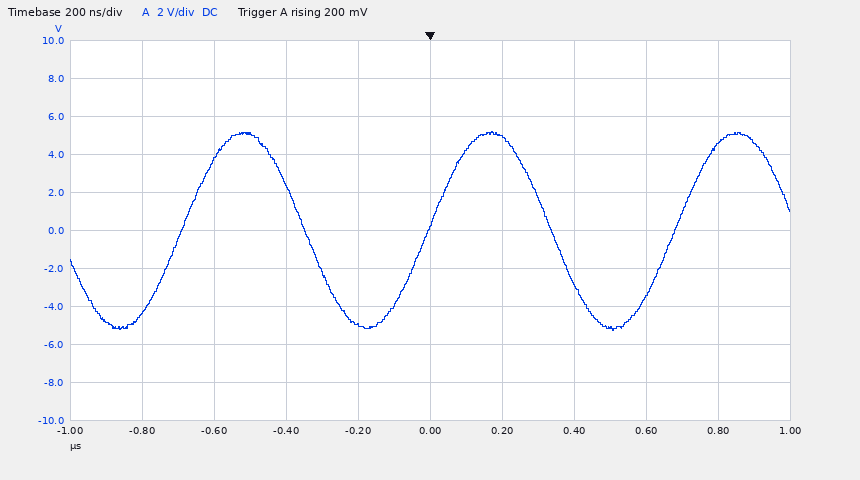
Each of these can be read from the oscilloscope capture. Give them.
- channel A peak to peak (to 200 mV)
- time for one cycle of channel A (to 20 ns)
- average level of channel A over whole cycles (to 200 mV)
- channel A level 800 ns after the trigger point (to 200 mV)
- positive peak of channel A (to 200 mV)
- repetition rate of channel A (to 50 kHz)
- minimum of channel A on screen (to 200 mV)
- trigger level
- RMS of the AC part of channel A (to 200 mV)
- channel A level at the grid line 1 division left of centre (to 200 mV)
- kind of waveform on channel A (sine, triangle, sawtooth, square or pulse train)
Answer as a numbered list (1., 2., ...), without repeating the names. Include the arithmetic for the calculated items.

1. 5.2 V − (-5.2 V) = 10.4 V
2. 680 ns
3. (5.2 V + (-5.2 V)) / 2 ≈ 0.0 V
4. 4.6 V
5. 5.2 V
6. 1 / 680 ns ≈ 1.47 MHz, so 1.45 MHz to the nearest 50 kHz
7. -5.2 V
8. 200 mV
9. 10.4 V / (2√2) ≈ 3.68 V, so 3.6 V to the nearest 200 mV
10. -5.0 V
11. sine
